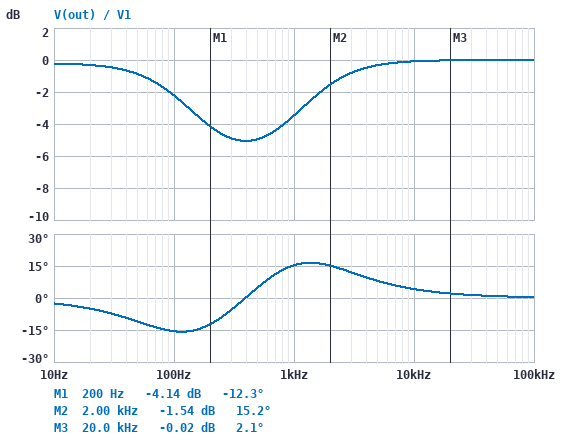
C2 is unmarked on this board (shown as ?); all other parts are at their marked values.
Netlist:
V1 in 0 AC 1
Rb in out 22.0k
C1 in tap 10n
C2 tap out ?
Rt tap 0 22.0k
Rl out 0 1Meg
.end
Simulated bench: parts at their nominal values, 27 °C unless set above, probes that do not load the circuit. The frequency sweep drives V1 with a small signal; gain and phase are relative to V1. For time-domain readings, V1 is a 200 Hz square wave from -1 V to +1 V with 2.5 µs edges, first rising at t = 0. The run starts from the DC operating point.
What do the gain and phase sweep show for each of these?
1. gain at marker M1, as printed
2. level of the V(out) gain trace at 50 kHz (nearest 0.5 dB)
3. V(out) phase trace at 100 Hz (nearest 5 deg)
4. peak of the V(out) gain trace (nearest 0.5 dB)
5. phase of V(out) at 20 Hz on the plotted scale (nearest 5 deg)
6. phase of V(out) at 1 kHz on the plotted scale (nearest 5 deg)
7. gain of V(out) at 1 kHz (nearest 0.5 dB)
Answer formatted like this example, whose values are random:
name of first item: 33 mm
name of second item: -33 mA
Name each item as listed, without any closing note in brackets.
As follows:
gain at marker M1, as printed: -4.14 dB
level of the V(out) gain trace at 50 kHz: 0 dB
V(out) phase trace at 100 Hz: -15 deg
peak of the V(out) gain trace: 0 dB
phase of V(out) at 20 Hz on the plotted scale: -5 deg
phase of V(out) at 1 kHz on the plotted scale: 15 deg
gain of V(out) at 1 kHz: -3.5 dB
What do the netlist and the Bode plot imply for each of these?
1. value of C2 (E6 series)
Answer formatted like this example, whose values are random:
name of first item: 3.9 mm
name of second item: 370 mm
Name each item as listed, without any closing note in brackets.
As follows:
value of C2: 33 nF
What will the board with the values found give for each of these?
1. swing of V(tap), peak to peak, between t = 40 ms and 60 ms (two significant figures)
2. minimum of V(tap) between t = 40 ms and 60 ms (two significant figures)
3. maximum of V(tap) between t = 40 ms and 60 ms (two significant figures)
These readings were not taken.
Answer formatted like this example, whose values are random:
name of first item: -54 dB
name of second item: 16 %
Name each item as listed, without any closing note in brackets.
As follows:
swing of V(tap), peak to peak, between t = 40 ms and 60 ms: 3.6 V
minimum of V(tap) between t = 40 ms and 60 ms: -1.8 V
maximum of V(tap) between t = 40 ms and 60 ms: 1.8 V
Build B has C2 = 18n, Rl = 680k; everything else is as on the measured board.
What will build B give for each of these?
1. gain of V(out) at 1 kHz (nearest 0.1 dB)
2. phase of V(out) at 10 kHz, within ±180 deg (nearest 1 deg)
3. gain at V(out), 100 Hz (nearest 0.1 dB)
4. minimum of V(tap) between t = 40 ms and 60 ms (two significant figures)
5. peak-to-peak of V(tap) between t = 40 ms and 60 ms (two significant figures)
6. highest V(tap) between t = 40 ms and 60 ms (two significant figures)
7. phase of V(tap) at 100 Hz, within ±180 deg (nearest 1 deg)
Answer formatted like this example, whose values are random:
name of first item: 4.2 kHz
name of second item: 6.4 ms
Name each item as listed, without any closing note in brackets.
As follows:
gain of V(out) at 1 kHz: -3.6 dB
phase of V(out) at 10 kHz, within ±180 deg: 4 deg
gain at V(out), 100 Hz: -1.2 dB
minimum of V(tap) between t = 40 ms and 60 ms: -1.9 V
peak-to-peak of V(tap) between t = 40 ms and 60 ms: 3.8 V
highest V(tap) between t = 40 ms and 60 ms: 1.9 V
phase of V(tap) at 100 Hz, within ±180 deg: 62 deg
